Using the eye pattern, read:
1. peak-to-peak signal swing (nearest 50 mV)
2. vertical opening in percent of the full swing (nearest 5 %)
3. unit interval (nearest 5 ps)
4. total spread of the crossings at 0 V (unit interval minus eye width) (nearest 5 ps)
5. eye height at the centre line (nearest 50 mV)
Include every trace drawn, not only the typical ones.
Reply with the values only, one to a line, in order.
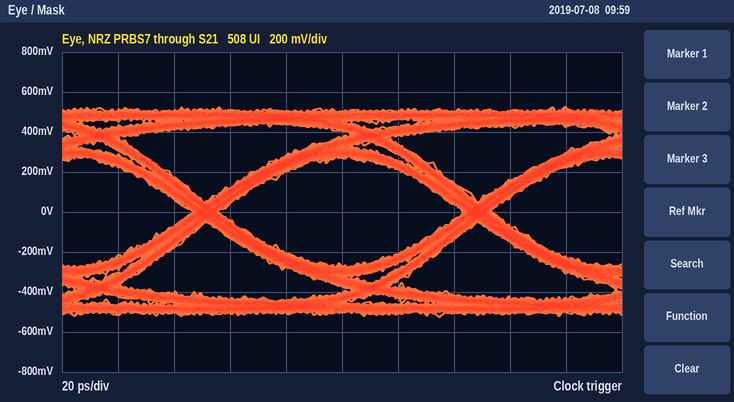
1.05 V
50 %
95 ps
10 ps
550 mV
